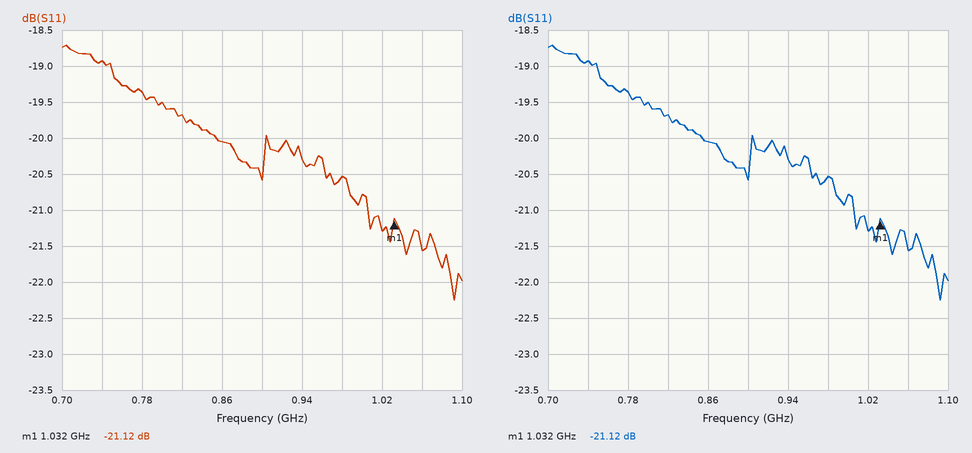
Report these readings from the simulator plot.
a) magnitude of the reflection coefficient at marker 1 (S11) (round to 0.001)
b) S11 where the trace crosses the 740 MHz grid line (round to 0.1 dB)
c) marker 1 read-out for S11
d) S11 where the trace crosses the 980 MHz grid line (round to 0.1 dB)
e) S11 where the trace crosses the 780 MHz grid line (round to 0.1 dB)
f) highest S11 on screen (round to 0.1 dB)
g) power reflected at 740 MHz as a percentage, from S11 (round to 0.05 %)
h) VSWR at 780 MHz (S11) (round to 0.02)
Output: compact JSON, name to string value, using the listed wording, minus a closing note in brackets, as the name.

{"magnitude of the reflection coefficient at marker 1 (S11)": "0.088", "S11 where the trace crosses the 740 MHz grid line": "-18.9 dB", "marker 1 read-out for S11": "-21.12 dB", "S11 where the trace crosses the 980 MHz grid line": "-20.5 dB", "S11 where the trace crosses the 780 MHz grid line": "-19.4 dB", "highest S11 on screen": "-18.7 dB", "power reflected at 740 MHz as a percentage, from S11": "1.30 %", "VSWR at 780 MHz (S11)": "1.24"}
